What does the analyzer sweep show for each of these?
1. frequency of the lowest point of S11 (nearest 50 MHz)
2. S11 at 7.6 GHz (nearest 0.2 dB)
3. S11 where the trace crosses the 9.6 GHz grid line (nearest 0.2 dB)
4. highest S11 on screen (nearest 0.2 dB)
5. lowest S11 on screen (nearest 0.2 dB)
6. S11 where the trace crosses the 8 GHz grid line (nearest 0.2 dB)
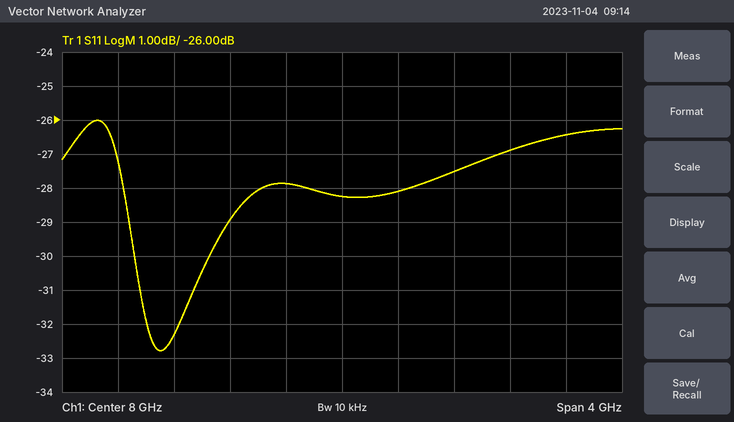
6.70 GHz
-27.8 dB
-26.4 dB
-26.0 dB
-32.8 dB
-28.2 dB
